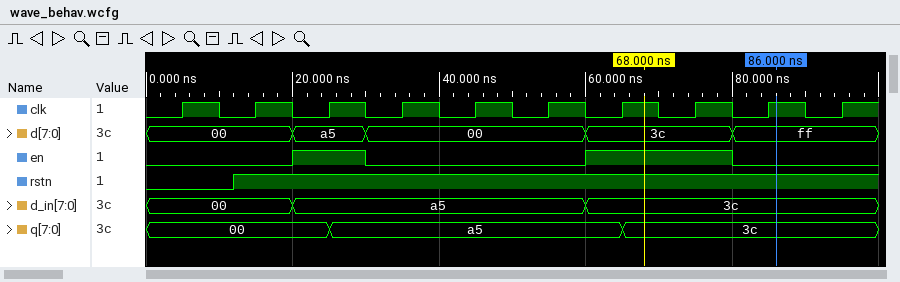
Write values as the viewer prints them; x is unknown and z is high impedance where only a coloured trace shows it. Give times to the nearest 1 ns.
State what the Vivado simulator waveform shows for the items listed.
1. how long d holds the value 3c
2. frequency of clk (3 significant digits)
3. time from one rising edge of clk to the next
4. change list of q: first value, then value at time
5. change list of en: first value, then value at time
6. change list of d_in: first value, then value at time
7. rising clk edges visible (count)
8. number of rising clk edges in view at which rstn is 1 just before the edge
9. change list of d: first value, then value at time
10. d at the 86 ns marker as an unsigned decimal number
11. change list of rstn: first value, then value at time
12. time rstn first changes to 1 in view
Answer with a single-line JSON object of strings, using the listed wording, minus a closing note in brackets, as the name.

{"how long d holds the value 3c": "20 ns", "frequency of clk": "100 MHz", "time from one rising edge of clk to the next": "10 ns", "change list of q: first value, then value at time": "00, a5 at 25 ns, 3c at 65 ns", "change list of en: first value, then value at time": "0, 1 at 20 ns, 0 at 30 ns, 1 at 60 ns, 0 at 80 ns", "change list of d_in: first value, then value at time": "00, a5 at 20 ns, 3c at 60 ns", "rising clk edges visible": "10", "number of rising clk edges in view at which rstn is 1 just before the edge": "9", "change list of d: first value, then value at time": "00, a5 at 20 ns, 00 at 30 ns, 3c at 60 ns, ff at 80 ns", "d at the 86 ns marker as an unsigned decimal number": "255", "change list of rstn: first value, then value at time": "0, 1 at 12 ns", "time rstn first changes to 1 in view": "12 ns"}
